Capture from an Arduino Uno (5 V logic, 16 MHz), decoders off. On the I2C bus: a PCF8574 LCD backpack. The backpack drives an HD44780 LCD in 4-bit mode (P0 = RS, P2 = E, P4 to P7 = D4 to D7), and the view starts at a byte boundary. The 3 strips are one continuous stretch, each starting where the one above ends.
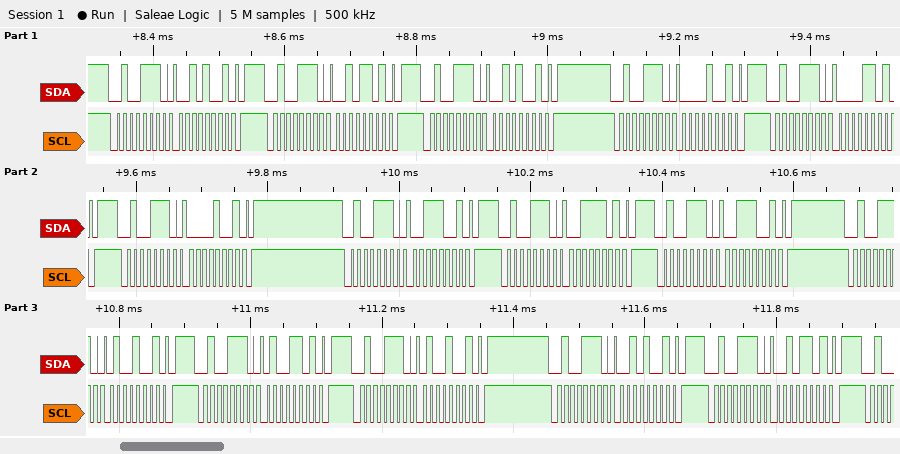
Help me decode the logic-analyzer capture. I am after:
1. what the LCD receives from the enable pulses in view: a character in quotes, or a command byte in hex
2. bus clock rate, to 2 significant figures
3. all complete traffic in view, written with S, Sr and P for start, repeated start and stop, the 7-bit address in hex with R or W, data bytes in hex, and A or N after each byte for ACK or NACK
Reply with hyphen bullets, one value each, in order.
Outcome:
- ' ' '4'
- 100 kHz
- S 27W A 29 A P S 27W A 2D A P S 27W A 29 A P S 27W A 09 A P S 27W A 0D A P S 27W A 09 A P S 27W A 39 A P S 27W A 3D A P S 27W A 39 A P S 27W A 49 A P S 27W A 4D A P S 27W A 49 A P S 27W A 29 A P S 27W A 2D A P
